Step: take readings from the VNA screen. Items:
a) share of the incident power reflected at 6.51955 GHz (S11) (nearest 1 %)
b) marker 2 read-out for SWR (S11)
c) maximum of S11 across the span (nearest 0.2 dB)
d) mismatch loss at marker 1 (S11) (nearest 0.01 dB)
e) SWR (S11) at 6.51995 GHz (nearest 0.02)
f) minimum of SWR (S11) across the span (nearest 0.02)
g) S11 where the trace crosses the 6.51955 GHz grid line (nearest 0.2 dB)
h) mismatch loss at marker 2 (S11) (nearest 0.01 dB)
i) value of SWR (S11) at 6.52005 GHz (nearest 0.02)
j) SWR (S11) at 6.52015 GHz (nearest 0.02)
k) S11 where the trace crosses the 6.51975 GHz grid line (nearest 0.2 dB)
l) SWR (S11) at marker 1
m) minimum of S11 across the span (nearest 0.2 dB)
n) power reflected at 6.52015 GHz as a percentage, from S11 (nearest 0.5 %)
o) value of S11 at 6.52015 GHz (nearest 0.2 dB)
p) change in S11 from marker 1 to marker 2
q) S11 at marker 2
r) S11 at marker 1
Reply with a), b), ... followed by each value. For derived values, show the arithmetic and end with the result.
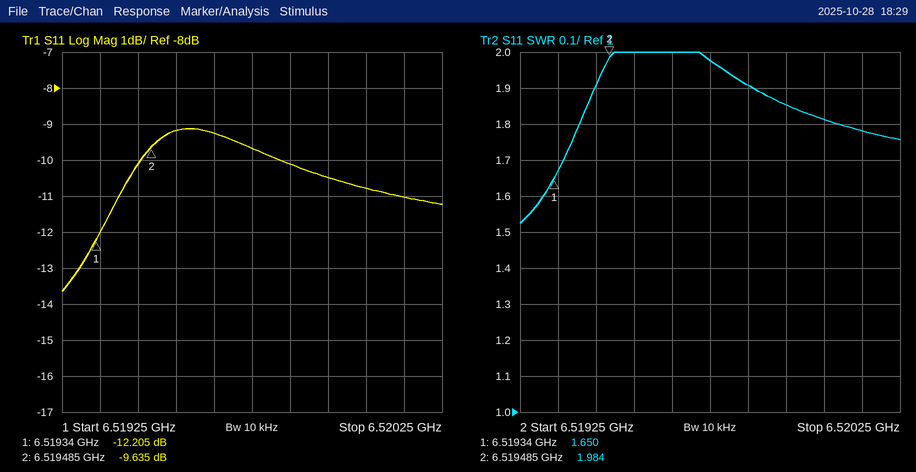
a) 10^(-9.2/10) ≈ 12 %
b) 1.984
c) -9.2 dB
d) −10 log10(1 − 10^(-12.205/10)) ≈ 0.27 dB
e) 1.86
f) 1.52
g) -9.2 dB
h) −10 log10(1 − 10^(-9.635/10)) ≈ 0.50 dB
i) 1.82
j) 1.78
k) -9.6 dB
l) 1.650
m) -13.6 dB
n) 10^(-11/10) ≈ 7.94 %, so 8.0 % to the nearest 0.5 %
o) -11.0 dB
p) -9.635 − (-12.205) = 2.570 dB
q) -9.635 dB
r) -12.205 dB
